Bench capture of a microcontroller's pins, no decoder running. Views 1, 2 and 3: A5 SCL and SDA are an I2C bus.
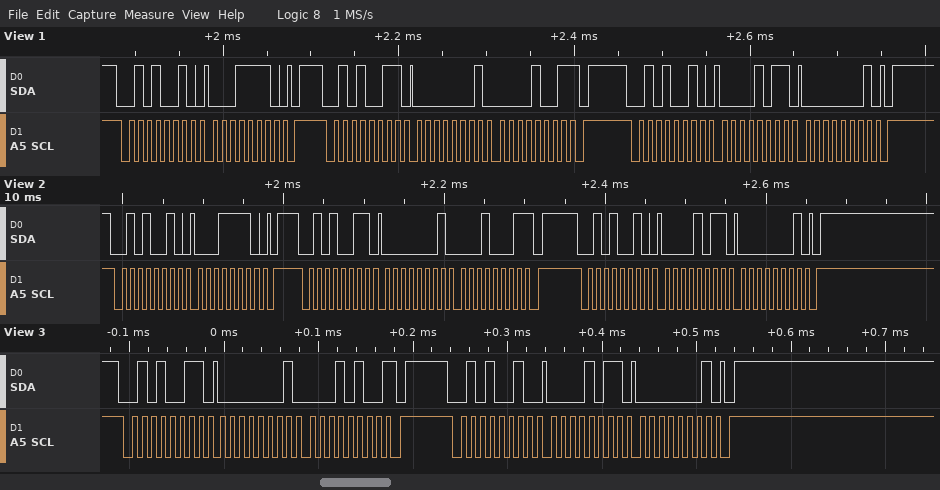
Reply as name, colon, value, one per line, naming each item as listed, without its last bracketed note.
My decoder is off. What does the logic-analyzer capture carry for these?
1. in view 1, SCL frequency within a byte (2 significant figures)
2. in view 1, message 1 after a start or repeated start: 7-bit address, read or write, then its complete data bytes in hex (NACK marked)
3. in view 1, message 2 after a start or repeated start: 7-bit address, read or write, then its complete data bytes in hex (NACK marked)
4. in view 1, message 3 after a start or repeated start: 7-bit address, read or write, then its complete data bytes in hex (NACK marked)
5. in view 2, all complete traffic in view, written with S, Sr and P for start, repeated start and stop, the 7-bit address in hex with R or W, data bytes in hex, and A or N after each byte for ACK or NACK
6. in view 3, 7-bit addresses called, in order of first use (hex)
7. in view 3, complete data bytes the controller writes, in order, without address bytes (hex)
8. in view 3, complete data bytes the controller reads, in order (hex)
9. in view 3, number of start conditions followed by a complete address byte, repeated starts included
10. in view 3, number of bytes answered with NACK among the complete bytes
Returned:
in view 1, SCL frequency within a byte: 100 kHz
in view 1, message 1 after a start or repeated start: 7-bit address, read or write, then its complete data bytes in hex: 0x29 write: 1E
in view 1, message 2 after a start or repeated start: 7-bit address, read or write, then its complete data bytes in hex: 0x29 read: 01 09 NACK
in view 1, message 3 after a start or repeated start: 7-bit address, read or write, then its complete data bytes in hex: 0x29 write: 0B 01
in view 2, all complete traffic in view, written with S, Sr and P for start, repeated start and stop, the 7-bit address in hex with R or W, data bytes in hex, and A or N after each byte for ACK or NACK: S 29W A 1E A P S 29R A 01 A 11 N P S 29W A 0B A 01 A P
in view 3, 7-bit addresses called, in order of first use: 0x29
in view 3, complete data bytes the controller writes, in order, without address bytes: 0B 01
in view 3, complete data bytes the controller reads, in order: 01 14
in view 3, number of start conditions followed by a complete address byte, repeated starts included: 2
in view 3, number of bytes answered with NACK among the complete bytes: 1
